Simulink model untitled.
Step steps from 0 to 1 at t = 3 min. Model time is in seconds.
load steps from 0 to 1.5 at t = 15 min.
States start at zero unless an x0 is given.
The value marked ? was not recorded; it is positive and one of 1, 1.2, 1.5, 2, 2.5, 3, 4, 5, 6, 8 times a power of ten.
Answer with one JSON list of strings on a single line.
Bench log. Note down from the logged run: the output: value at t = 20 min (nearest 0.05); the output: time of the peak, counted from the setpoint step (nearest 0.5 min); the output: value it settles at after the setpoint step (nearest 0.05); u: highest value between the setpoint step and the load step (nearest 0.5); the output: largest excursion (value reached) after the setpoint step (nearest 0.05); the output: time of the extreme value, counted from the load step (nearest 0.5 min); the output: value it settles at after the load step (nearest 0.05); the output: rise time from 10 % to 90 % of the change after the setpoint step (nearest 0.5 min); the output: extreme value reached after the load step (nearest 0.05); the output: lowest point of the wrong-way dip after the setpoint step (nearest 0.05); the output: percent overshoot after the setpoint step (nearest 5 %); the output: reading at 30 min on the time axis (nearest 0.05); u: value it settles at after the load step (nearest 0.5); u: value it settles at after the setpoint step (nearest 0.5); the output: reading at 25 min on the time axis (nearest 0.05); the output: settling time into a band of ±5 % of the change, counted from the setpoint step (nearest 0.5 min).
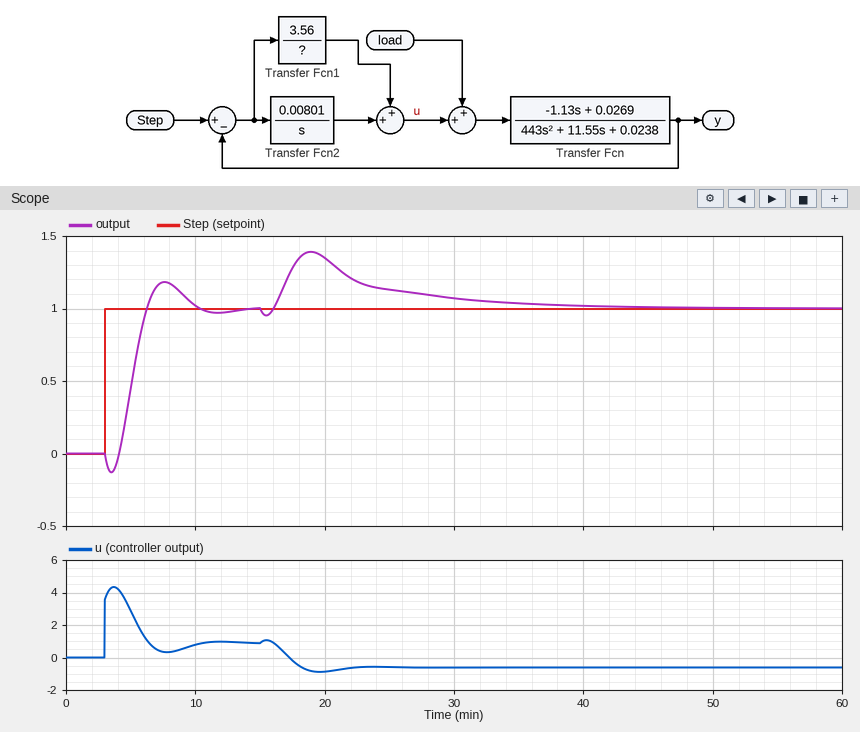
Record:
["1.35", "4.5 min", "1.00", "4.5", "1.20", "4.0 min", "1.00", "1.5 min", "1.40", "-0.15", "20 %", "1.05", "-0.5", "1.0", "1.15", "6.5 min"]
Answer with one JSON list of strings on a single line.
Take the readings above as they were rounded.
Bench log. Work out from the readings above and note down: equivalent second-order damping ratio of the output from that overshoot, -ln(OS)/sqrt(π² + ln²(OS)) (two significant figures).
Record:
["0.46"]
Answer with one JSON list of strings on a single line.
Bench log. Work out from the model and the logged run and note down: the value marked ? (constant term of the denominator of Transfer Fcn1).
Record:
["1"]
